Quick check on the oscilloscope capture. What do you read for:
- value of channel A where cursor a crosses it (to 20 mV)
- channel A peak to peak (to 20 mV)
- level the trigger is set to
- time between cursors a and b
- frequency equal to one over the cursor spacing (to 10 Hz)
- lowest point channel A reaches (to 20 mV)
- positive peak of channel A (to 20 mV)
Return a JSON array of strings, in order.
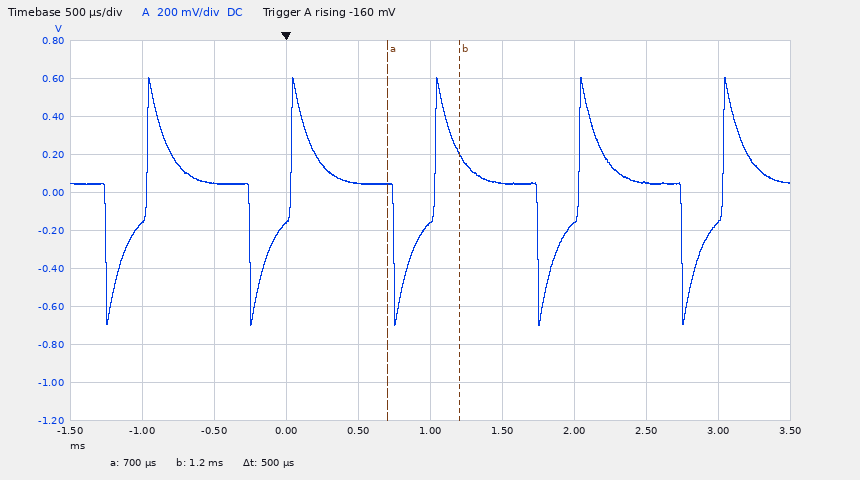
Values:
["40 mV", "1.30 V", "-160 mV", "500 µs", "2.00 kHz", "-700 mV", "600 mV"]
